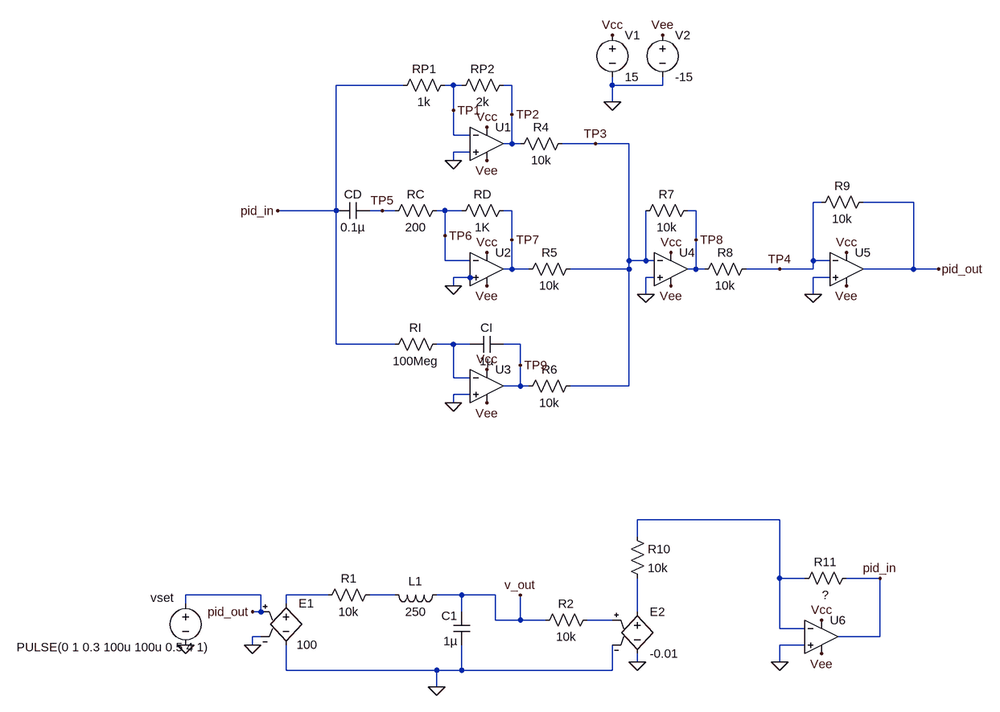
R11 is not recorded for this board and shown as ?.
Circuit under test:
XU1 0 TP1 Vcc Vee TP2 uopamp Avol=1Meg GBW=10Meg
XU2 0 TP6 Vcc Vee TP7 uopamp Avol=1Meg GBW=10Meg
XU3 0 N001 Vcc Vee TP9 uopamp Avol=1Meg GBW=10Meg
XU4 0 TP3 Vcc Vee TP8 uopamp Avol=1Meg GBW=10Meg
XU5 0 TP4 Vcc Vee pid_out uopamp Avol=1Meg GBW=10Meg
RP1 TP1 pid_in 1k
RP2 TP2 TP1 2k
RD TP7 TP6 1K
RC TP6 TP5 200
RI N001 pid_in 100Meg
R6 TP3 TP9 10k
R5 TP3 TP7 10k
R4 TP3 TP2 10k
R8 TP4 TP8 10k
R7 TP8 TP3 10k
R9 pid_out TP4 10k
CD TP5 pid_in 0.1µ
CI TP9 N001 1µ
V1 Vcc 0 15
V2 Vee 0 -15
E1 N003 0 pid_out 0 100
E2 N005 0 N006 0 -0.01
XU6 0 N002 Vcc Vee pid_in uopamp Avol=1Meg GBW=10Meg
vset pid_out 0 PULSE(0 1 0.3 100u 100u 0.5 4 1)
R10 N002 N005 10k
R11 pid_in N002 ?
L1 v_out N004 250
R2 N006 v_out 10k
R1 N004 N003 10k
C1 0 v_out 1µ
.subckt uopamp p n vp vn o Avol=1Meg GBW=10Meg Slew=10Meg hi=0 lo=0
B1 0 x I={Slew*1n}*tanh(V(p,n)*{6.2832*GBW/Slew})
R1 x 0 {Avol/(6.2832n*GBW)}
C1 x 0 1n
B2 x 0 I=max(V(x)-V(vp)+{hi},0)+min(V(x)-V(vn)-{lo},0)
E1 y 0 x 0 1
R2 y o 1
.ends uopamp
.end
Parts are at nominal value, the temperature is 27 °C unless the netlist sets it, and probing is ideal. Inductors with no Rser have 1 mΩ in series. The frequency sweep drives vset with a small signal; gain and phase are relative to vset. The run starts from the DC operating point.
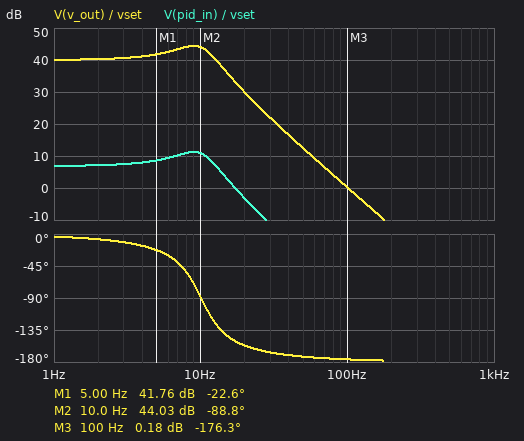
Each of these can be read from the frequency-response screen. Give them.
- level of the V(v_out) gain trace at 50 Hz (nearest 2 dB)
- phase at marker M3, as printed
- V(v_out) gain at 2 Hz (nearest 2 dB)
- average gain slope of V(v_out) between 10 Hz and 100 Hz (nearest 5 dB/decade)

12 dB
-176.3 deg
40 dB
-45 dB/decade
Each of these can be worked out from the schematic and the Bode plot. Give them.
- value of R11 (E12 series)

22 kΩ
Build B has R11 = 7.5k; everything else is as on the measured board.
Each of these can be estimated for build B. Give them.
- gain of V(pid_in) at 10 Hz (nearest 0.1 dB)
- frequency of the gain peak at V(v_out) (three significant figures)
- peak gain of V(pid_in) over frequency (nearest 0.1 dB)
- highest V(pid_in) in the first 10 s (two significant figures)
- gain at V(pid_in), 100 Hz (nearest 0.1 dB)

1.5 dB
9.00 Hz
1.9 dB
1.0 V
-42.3 dB
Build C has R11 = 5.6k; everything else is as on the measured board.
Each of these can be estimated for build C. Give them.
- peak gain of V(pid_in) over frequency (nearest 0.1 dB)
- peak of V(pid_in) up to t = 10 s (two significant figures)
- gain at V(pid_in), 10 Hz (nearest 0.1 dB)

-0.6 dB
760 mV
-1.0 dB
